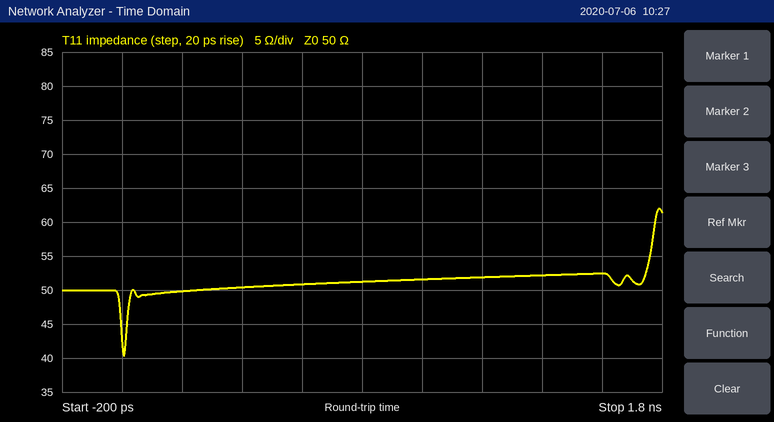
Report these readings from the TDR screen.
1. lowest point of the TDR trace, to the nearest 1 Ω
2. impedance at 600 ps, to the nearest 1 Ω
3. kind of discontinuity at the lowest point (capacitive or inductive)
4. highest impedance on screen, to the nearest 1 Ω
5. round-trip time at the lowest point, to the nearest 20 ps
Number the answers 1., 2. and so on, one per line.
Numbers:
1. 40 Ω
2. 51 Ω
3. capacitive
4. 62 Ω
5. 0 ps
